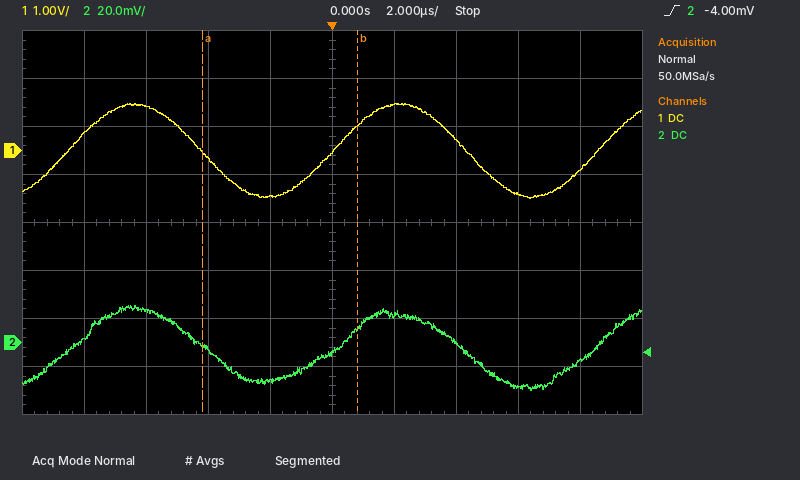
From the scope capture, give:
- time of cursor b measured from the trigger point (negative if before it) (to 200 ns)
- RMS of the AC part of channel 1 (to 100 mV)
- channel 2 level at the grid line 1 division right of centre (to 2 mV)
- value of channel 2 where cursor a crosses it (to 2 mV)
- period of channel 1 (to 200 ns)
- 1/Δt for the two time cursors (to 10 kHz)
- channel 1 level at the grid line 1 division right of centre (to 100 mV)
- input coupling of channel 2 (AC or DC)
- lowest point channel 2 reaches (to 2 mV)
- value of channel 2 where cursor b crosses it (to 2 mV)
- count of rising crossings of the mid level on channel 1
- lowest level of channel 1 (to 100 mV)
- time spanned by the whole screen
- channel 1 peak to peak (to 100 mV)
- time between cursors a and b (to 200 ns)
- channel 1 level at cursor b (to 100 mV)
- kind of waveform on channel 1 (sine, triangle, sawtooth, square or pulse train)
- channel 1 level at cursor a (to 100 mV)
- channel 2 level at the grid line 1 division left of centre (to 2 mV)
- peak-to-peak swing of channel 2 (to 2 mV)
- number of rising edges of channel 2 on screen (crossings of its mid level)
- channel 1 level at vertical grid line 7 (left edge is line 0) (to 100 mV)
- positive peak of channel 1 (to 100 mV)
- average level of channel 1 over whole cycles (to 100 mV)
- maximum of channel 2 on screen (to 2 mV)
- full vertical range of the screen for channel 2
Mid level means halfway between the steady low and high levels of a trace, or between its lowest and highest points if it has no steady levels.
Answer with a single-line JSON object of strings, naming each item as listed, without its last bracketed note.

{"time of cursor b measured from the trigger point (negative if before it)": "+800 ns", "RMS of the AC part of channel 1": "700 mV", "channel 2 level at the grid line 1 division right of centre": "12 mV", "value of channel 2 where cursor a crosses it": "-2 mV", "period of channel 1": "8.6 µs", "1/Δt for the two time cursors": "200 kHz", "channel 1 level at the grid line 1 division right of centre": "1.0 V", "input coupling of channel 2": "DC", "lowest point channel 2 reaches": "-20 mV", "value of channel 2 where cursor b crosses it": "6 mV", "count of rising crossings of the mid level on channel 1": "3", "lowest level of channel 1": "-1.0 V", "time spanned by the whole screen": "20 µs", "channel 1 peak to peak": "2.0 V", "time between cursors a and b": "5.0 µs", "channel 1 level at cursor b": "500 mV", "kind of waveform on channel 1": "sine", "channel 1 level at cursor a": "0.0 V", "channel 2 level at the grid line 1 division left of centre": "-16 mV", "peak-to-peak swing of channel 2": "36 mV", "number of rising edges of channel 2 on screen": "3", "channel 1 level at vertical grid line 7 (left edge is line 0)": "200 mV", "positive peak of channel 1": "1.0 V", "average level of channel 1 over whole cycles": "0.0 V", "maximum of channel 2 on screen": "16 mV", "full vertical range of the screen for channel 2": "160 mV"}
